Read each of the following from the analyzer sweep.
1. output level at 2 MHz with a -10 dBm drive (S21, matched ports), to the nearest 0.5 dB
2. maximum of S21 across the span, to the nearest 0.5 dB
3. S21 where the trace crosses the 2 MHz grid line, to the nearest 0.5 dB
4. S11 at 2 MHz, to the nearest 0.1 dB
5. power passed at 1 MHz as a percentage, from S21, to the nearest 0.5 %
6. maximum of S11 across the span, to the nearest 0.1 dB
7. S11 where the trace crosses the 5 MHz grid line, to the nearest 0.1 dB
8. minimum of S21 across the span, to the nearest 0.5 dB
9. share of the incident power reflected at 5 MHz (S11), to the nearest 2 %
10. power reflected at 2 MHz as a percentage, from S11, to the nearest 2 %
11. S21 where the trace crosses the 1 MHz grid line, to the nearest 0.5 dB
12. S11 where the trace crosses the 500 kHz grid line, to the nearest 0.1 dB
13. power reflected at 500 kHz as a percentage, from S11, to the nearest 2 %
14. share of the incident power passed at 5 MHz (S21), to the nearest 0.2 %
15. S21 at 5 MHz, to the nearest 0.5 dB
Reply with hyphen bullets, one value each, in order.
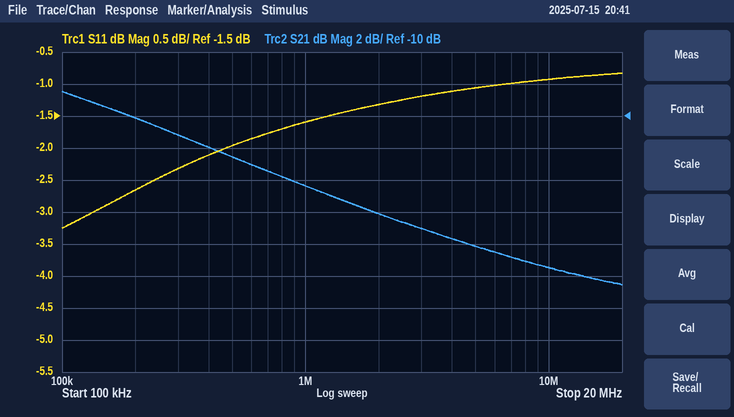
- -26.0 dBm
- -8.5 dB
- -16.0 dB
- -1.3 dB
- 3.5 %
- -0.8 dB
- -1.1 dB
- -20.5 dB
- 78 %
- 74 %
- -14.5 dB
- -2.0 dB
- 64 %
- 1.6 %
- -18.0 dB
